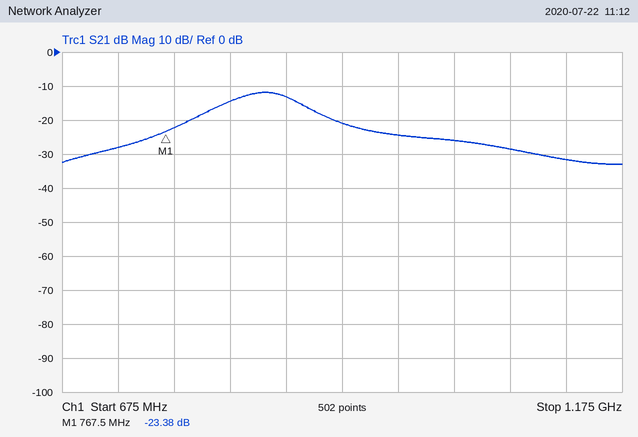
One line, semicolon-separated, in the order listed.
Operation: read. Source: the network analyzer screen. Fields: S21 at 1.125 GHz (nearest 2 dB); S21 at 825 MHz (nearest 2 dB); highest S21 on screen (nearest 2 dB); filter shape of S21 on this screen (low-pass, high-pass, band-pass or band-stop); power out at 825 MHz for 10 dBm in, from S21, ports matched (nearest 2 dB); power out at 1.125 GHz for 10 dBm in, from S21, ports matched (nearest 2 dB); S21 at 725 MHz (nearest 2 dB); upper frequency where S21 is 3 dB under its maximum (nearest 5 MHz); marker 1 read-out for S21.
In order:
-32 dB; -14 dB; -12 dB; band-pass; -4 dBm; -22 dBm; -28 dB; 885 MHz; -23.38 dB
